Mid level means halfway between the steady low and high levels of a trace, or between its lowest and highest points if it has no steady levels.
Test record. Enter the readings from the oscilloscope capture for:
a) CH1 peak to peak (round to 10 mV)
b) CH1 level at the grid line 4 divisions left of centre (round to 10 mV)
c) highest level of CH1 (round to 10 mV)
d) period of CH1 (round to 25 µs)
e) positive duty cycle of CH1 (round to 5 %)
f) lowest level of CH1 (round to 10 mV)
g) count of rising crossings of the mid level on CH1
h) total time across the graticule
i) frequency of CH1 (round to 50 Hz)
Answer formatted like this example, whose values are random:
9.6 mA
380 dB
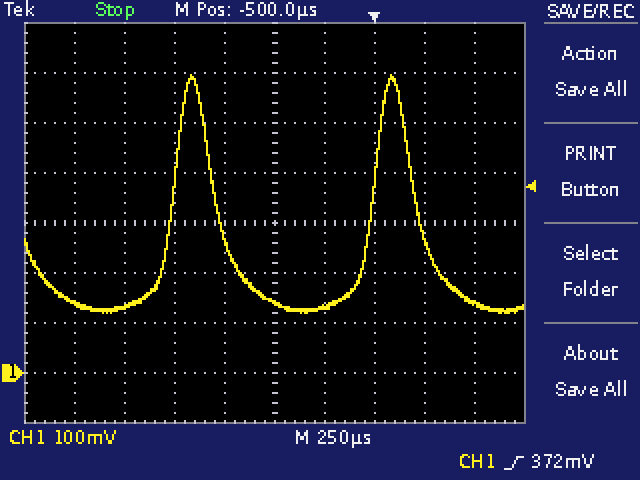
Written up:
480 mV
140 mV
600 mV
1.000 ms
20 %
120 mV
2
2.5 ms
1.00 kHz
